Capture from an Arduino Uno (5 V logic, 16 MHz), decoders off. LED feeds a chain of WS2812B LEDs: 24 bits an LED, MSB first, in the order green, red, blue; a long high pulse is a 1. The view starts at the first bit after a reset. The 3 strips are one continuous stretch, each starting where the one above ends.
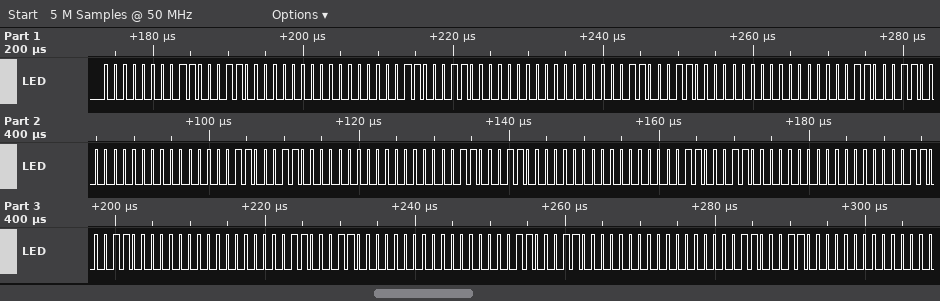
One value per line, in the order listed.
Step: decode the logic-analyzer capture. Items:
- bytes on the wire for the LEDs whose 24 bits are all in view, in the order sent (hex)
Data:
00 C6 00 00 C6 00 00 C6 00 00 C6 00 00 C6 00 00 C6 00 00 C6 00 00 C6 00 00 C6 00 00 C6 00 00 C6 00
